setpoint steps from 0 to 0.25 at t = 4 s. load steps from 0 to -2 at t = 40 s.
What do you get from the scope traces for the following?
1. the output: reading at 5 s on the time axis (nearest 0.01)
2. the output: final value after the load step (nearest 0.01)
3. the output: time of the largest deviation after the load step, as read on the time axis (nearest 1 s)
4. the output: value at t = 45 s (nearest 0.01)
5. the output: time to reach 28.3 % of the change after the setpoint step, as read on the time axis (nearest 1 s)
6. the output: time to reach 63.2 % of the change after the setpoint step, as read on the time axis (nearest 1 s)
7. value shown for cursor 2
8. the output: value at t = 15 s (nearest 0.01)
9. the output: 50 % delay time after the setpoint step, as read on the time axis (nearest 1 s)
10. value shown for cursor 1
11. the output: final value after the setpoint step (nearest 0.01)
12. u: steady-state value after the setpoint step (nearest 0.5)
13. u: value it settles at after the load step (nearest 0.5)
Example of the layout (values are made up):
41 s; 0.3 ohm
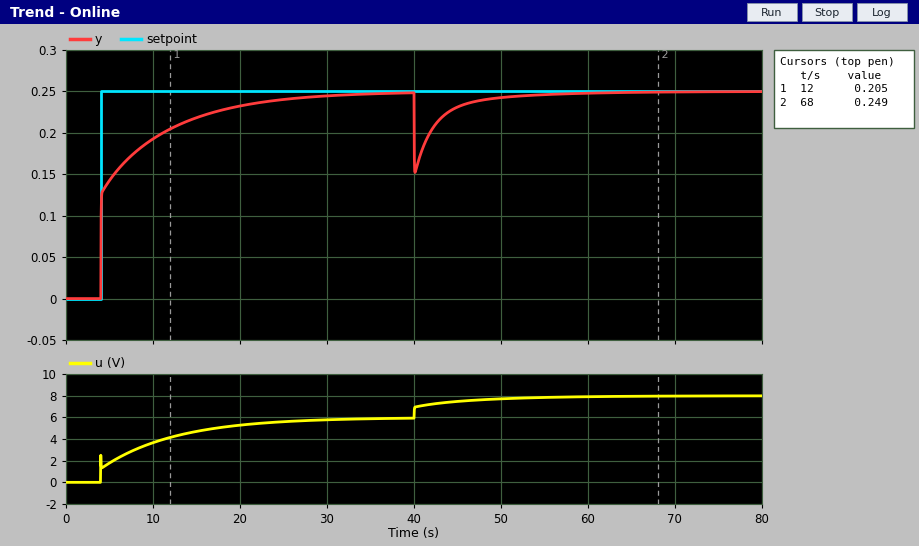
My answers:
0.14; 0.25; 40 s; 0.23; 4 s; 6 s; 0.249; 0.22; 4 s; 0.205; 0.25; 6.0; 8.0
